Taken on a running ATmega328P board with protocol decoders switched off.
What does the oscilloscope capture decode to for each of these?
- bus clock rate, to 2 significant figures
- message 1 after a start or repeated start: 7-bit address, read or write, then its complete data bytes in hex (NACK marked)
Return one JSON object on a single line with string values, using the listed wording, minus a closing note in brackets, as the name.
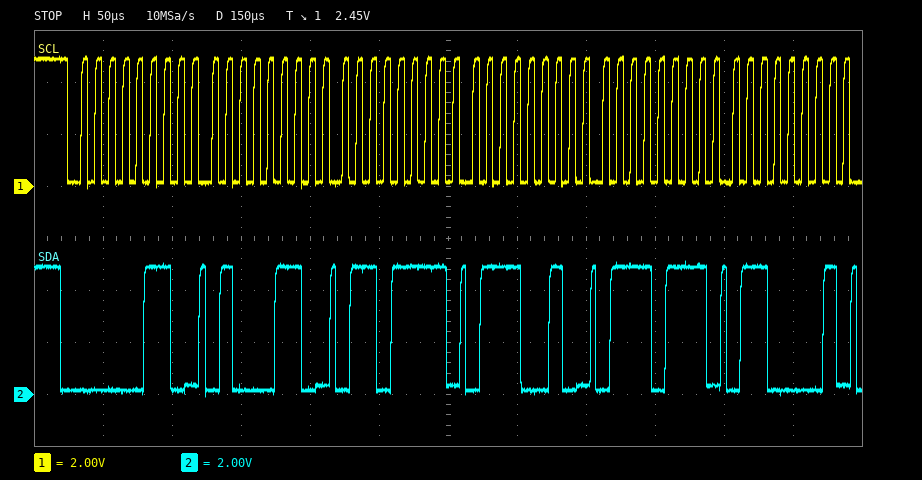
{"bus clock rate, to 2 significant figures": "100 kHz", "message 1 after a start or repeated start: 7-bit address, read or write, then its complete data bytes in hex": "0x03 write: 46 6F 72 77 61"}
